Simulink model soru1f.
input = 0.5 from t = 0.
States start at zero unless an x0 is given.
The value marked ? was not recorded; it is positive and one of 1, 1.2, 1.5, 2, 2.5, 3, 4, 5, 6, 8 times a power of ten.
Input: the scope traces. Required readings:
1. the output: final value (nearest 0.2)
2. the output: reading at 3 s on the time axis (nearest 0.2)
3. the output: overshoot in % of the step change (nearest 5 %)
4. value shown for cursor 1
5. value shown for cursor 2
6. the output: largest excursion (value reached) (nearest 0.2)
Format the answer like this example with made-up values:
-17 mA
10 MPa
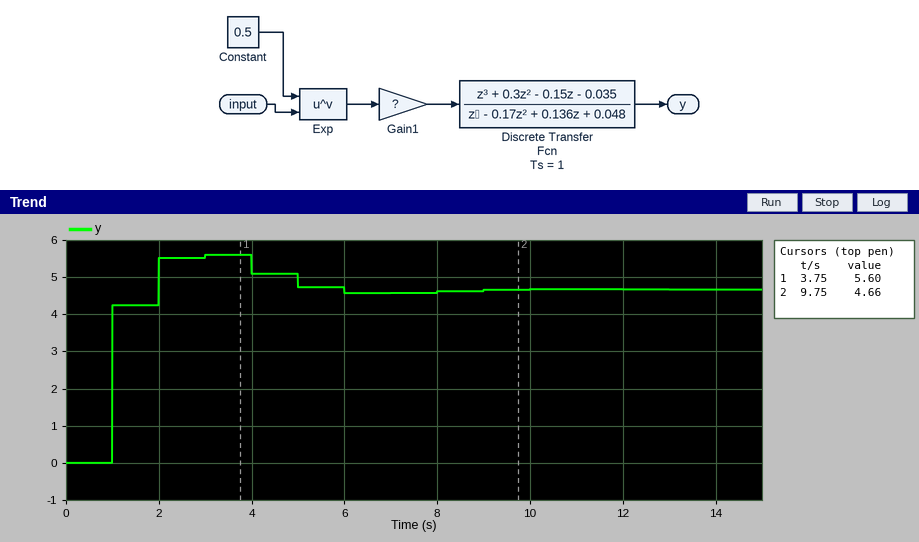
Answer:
4.6
5.6
20 %
5.60
4.66
5.6
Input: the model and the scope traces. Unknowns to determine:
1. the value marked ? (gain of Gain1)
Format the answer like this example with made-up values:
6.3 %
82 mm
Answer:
6
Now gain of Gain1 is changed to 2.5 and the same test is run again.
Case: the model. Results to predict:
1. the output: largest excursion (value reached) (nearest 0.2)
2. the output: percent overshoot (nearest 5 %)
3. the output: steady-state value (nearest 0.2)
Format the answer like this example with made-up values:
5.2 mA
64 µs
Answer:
2.4
20 %
2.0
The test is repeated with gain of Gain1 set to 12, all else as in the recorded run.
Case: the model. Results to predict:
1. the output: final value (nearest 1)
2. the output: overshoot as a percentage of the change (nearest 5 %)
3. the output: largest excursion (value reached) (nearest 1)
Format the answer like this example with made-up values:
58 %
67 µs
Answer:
9
20 %
11
